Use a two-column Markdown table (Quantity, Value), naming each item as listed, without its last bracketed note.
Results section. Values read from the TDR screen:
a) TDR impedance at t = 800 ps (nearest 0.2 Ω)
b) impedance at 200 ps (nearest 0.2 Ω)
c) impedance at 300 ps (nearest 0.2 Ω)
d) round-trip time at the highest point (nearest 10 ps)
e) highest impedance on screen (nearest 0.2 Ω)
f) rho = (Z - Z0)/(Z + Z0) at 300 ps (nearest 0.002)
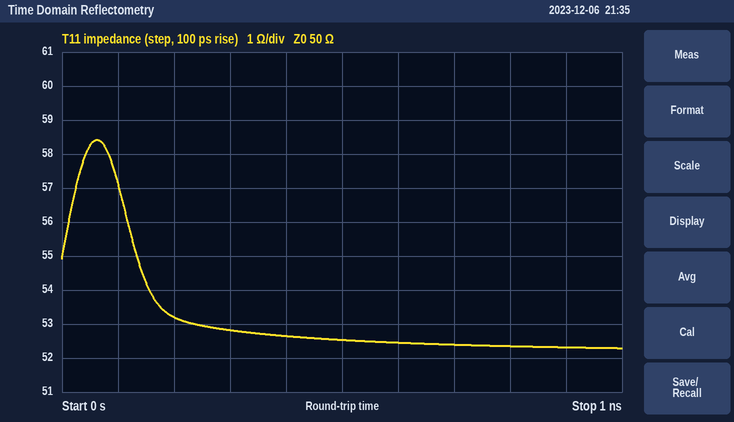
| Quantity | Value |
|---|---|
| TDR impedance at t = 800 ps | 52.4 Ω |
| impedance at 200 ps | 53.2 Ω |
| impedance at 300 ps | 52.8 Ω |
| round-trip time at the highest point | 60 ps |
| highest impedance on screen | 58.4 Ω |
| rho = (Z - Z0)/(Z + Z0) at 300 ps | +0.028 |
